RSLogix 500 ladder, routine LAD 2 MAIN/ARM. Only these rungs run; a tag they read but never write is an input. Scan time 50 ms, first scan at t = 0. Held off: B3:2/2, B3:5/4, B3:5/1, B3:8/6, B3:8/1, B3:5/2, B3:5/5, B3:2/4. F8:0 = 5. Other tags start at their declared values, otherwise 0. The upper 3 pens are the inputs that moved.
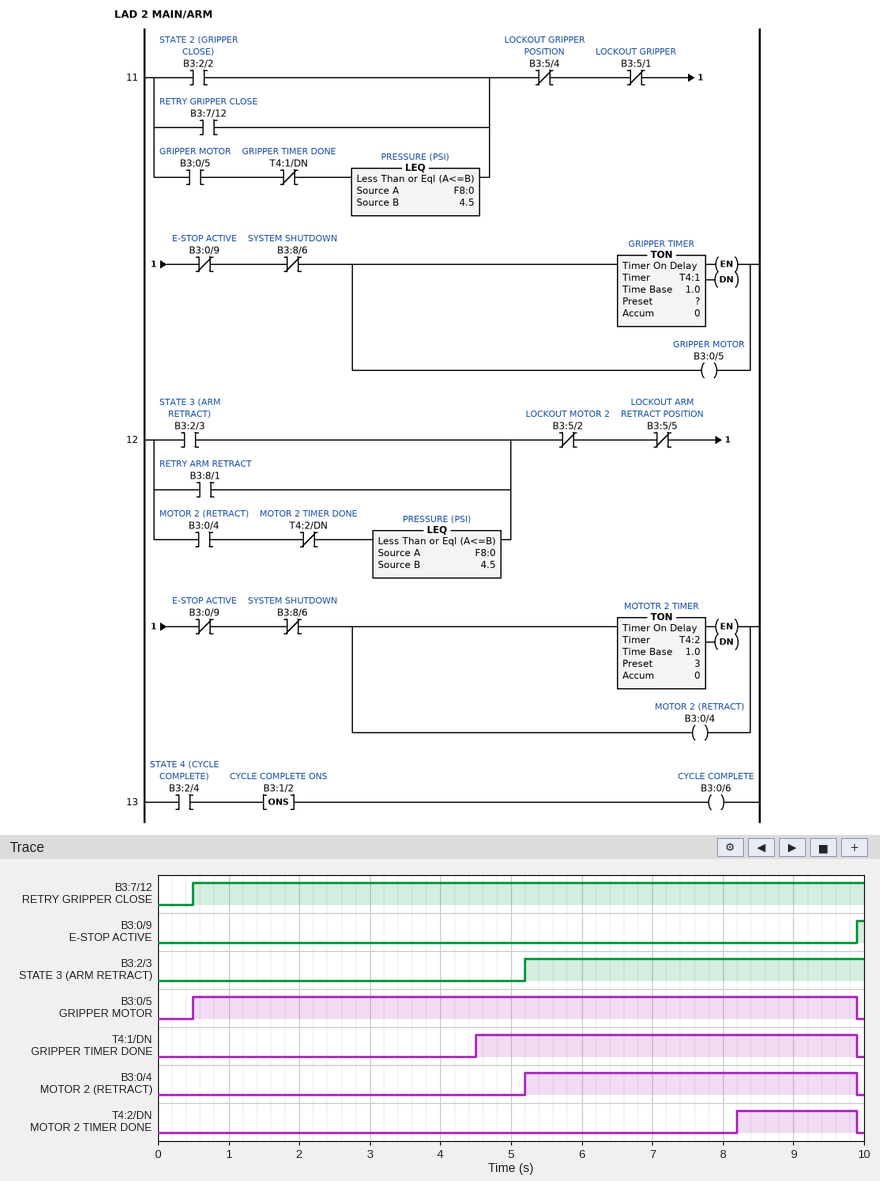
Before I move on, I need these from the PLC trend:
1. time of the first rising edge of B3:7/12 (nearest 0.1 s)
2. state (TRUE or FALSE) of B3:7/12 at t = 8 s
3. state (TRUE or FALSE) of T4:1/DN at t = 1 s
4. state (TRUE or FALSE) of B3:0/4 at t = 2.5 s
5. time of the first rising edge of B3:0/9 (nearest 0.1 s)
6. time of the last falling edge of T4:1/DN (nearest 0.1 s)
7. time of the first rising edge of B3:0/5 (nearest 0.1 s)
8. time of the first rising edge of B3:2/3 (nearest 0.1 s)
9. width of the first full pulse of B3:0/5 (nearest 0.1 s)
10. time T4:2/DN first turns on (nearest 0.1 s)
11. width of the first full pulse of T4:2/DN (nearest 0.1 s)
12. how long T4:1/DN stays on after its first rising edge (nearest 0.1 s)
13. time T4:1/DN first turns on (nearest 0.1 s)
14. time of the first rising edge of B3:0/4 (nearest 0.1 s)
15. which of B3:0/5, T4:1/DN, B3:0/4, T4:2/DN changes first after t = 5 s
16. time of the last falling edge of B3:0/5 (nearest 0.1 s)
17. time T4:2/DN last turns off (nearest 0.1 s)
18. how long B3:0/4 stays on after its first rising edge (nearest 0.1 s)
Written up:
0.5 s
TRUE
FALSE
FALSE
9.9 s
9.9 s
0.5 s
5.2 s
9.4 s
8.2 s
1.7 s
5.4 s
4.5 s
5.2 s
B3:0/4
9.9 s
9.9 s
4.7 s
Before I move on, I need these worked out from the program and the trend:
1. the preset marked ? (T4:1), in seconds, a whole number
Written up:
4 s
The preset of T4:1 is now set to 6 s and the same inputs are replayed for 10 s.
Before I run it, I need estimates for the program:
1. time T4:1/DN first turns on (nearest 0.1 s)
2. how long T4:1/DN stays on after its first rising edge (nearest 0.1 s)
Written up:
6.5 s
3.4 s
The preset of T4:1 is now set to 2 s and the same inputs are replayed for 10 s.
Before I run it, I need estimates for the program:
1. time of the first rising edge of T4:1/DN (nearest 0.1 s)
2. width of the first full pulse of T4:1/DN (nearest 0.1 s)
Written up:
2.5 s
7.4 s
